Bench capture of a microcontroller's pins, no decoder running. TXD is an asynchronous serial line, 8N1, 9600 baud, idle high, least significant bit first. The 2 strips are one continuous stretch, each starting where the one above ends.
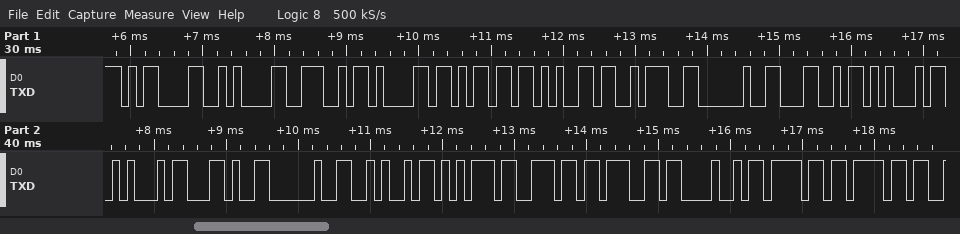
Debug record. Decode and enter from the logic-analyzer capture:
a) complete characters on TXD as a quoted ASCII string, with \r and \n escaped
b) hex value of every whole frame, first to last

"\r\nName: LEE, JungHoo"
0D 0A 4E 61 6D 65 3A 20 4C 45 45 2C 20 4A 75 6E 67 48 6F 6F
